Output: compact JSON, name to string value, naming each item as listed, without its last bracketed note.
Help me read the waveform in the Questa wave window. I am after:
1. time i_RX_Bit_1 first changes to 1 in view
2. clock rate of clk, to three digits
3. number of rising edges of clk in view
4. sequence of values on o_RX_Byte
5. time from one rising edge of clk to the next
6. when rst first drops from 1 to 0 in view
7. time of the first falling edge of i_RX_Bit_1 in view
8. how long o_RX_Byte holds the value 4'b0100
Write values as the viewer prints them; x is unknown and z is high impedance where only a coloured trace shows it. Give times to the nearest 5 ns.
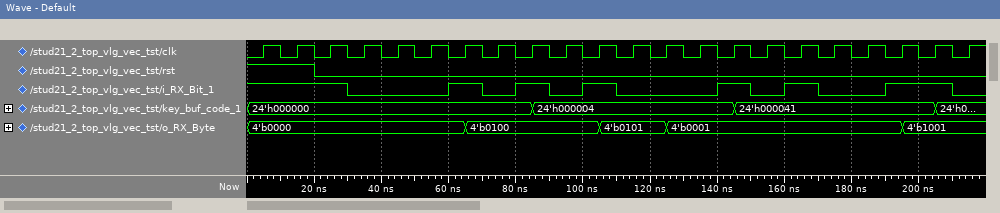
{"time i_RX_Bit_1 first changes to 1 in view": "60 ns", "clock rate of clk, to three digits": "100 MHz", "number of rising edges of clk in view": "22", "sequence of values on o_RX_Byte": "4'b0000, 4'b0100, 4'b0101, 4'b0001, 4'b1001", "time from one rising edge of clk to the next": "10 ns", "when rst first drops from 1 to 0 in view": "20 ns", "time of the first falling edge of i_RX_Bit_1 in view": "30 ns", "how long o_RX_Byte holds the value 4'b0100": "40 ns"}
